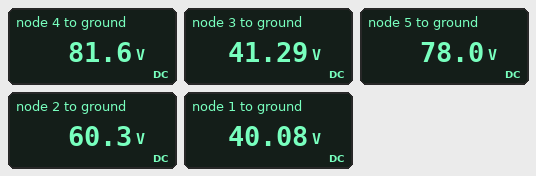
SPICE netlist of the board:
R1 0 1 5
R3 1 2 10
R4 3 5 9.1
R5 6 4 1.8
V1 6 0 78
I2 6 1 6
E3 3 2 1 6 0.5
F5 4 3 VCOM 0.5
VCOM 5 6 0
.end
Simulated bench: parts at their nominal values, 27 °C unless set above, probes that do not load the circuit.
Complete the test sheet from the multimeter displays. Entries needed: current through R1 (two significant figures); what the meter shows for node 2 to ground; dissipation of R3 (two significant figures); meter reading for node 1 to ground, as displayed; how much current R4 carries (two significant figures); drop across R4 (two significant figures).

8.0 A
60.3 V
41 W
40.08 V
4.0 A
37 V
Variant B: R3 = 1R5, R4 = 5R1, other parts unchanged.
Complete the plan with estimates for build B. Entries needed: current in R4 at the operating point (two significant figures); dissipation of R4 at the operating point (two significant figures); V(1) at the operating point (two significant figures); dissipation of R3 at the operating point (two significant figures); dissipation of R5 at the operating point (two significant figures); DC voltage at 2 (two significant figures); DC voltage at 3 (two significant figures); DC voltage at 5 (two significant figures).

7.5 A
290 W
49 V
21 W
25 W
54 V
40 V
78 V
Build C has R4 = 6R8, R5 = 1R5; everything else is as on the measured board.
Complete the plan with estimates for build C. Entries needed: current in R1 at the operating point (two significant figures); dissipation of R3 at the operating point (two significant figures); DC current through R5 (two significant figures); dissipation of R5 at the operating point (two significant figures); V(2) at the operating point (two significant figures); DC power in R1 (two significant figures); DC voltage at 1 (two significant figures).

8.3 A
54 W
2.3 A
8.0 W
65 V
350 W
42 V
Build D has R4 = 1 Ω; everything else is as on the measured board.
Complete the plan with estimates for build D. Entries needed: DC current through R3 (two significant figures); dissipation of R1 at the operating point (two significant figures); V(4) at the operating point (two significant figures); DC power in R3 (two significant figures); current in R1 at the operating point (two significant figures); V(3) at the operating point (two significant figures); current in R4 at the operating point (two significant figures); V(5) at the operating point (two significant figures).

3.7 A
470 W
85 V
140 W
9.7 A
71 V
7.4 A
78 V
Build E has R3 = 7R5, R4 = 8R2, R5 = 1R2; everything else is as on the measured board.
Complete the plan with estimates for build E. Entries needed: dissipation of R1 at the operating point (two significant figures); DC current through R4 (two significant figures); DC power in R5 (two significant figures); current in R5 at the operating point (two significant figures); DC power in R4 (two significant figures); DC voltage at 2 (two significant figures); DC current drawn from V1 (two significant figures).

340 W
4.6 A
6.3 W
2.3 A
170 W
59 V
8.3 A
